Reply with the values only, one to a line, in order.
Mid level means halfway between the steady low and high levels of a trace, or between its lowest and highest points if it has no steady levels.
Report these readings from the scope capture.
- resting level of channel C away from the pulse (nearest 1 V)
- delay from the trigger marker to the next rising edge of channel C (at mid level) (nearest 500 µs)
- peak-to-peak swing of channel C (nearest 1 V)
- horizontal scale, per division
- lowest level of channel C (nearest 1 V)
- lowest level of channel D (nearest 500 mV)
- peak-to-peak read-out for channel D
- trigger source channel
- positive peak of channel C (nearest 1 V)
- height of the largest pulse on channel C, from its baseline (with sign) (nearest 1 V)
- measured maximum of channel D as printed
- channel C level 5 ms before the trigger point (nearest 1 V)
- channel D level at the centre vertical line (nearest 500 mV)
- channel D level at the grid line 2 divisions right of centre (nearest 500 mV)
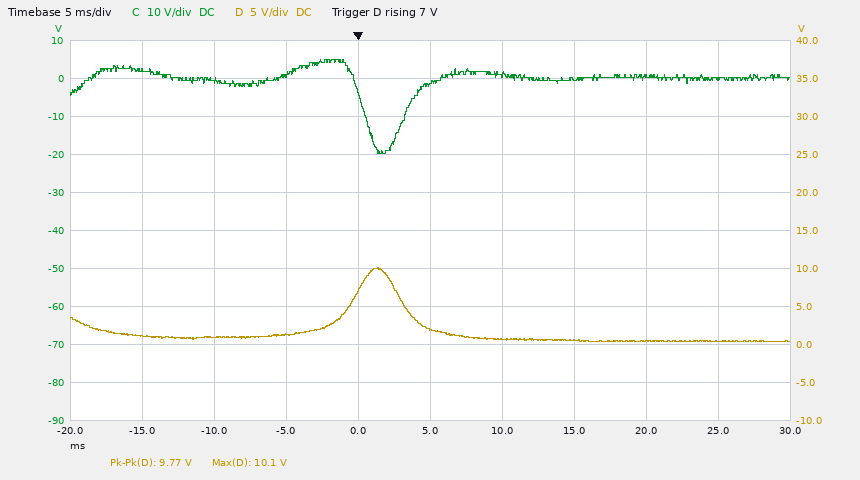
0 V
3.5 ms
25 V
5 ms
-20 V
500 mV
9.77 V
channel D
5 V
-20 V
10.1 V
1 V
2.0 V
500 mV
